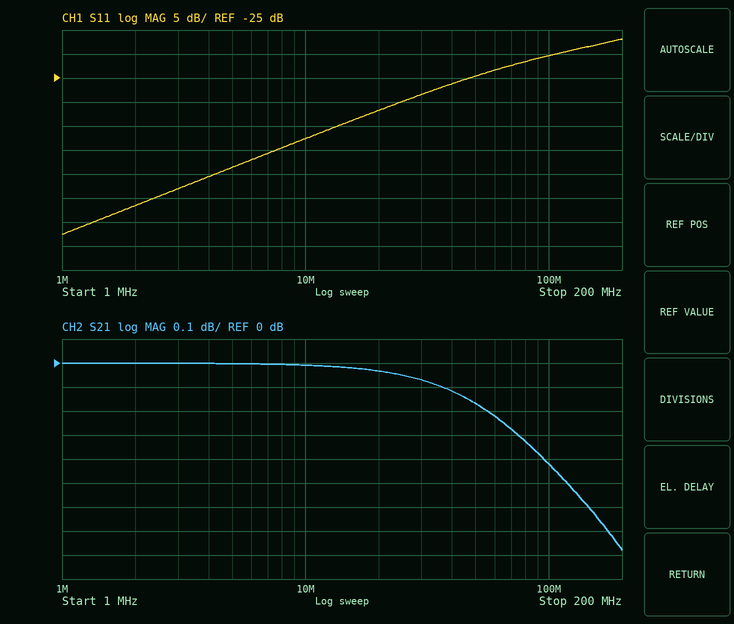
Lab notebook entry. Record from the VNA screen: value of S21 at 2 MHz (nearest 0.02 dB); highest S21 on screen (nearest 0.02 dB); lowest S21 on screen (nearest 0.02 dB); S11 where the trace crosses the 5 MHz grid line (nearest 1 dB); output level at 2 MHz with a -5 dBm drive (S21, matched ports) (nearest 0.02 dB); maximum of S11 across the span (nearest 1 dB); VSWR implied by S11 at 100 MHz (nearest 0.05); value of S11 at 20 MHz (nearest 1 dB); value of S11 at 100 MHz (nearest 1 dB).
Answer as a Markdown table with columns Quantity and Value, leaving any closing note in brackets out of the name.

| Quantity | Value |
|---|---|
| value of S21 at 2 MHz | 0.00 dB |
| highest S21 on screen | 0.00 dB |
| lowest S21 on screen | -0.78 dB |
| S11 where the trace crosses the 5 MHz grid line | -44 dB |
| output level at 2 MHz with a -5 dBm drive (S21, matched ports) | -5.00 dBm |
| maximum of S11 across the span | -17 dB |
| VSWR implied by S11 at 100 MHz | 1.20 |
| value of S11 at 20 MHz | -32 dB |
| value of S11 at 100 MHz | -20 dB |
